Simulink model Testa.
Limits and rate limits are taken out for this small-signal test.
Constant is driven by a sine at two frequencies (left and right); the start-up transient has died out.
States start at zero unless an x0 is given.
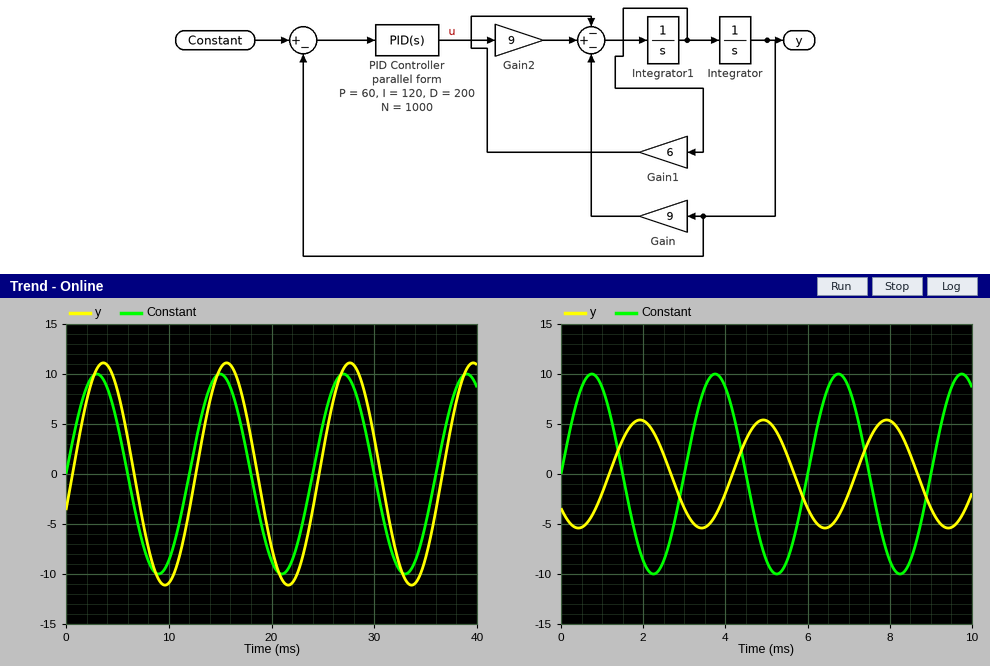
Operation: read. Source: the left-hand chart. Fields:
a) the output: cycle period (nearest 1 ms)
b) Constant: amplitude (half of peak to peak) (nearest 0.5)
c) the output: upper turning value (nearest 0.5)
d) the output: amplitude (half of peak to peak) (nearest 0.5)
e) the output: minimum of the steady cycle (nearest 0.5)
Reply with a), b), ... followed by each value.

a) 12 ms
b) 10.0
c) 11.0
d) 11.0
e) -11.0
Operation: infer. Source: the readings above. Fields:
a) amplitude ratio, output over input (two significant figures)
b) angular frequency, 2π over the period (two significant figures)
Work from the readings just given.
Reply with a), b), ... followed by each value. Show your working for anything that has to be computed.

a) 11 / 10 = 1.1
b) 2π / 12 = 0.52 rad/ms
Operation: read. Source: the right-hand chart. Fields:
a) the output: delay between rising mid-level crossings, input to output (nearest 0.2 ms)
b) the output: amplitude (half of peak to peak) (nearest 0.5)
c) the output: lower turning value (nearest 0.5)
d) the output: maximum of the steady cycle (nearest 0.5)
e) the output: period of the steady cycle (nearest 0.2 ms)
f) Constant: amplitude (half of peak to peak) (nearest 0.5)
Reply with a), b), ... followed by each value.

a) 1.2 ms
b) 5.5
c) -5.5
d) 5.5
e) 3.0 ms
f) 10.0
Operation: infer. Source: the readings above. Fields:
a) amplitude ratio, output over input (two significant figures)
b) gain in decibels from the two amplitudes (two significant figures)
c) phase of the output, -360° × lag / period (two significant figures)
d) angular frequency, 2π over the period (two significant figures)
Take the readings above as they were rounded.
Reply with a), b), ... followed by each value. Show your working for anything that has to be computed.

a) 5.5 / 10 = 0.55
b) 20 log10(5.5 / 10) = -5.2 dB
c) -360 × 1.2 / 3 = -140°
d) 2π / 3 = 2.1 rad/ms
